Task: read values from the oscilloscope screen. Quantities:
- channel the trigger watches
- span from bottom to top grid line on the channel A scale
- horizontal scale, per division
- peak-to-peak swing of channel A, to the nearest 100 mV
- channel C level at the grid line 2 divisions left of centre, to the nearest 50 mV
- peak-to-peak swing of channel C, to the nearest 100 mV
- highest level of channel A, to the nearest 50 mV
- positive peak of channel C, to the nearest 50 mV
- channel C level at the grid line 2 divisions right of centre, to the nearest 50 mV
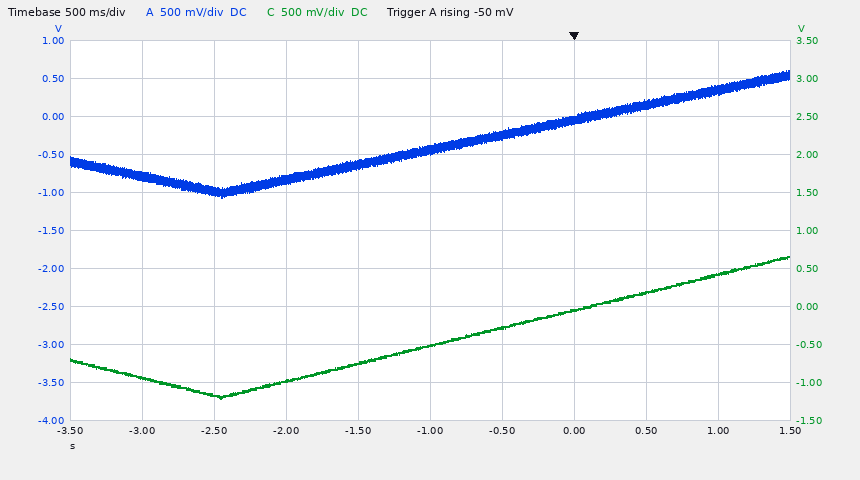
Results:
channel A
5 V
500 ms
1.70 V
-1.00 V
1.90 V
600 mV
650 mV
-50 mV
